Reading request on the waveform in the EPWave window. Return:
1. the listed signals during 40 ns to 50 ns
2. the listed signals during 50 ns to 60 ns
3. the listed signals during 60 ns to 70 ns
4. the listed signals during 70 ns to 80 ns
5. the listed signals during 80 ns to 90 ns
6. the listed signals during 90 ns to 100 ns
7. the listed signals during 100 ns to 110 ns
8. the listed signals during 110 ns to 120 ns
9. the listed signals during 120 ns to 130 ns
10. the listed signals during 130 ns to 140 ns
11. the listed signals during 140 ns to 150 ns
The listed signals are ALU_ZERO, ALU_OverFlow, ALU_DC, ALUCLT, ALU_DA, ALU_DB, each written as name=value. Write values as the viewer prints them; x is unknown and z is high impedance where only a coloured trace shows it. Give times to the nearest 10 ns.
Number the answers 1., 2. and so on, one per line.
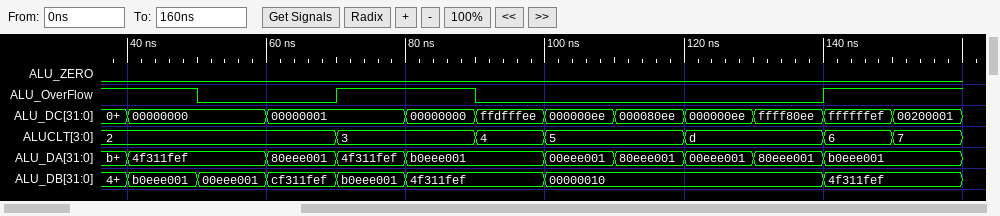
1. ALU_ZERO=0, ALU_OverFlow=1, ALU_DC=00000000, ALUCLT=2, ALU_DA=4f311fef, ALU_DB=b0eee001
2. ALU_ZERO=0, ALU_OverFlow=0, ALU_DC=00000000, ALUCLT=2, ALU_DA=4f311fef, ALU_DB=00eee001
3. ALU_ZERO=0, ALU_OverFlow=0, ALU_DC=00000001, ALUCLT=2, ALU_DA=80eee001, ALU_DB=cf311fef
4. ALU_ZERO=0, ALU_OverFlow=1, ALU_DC=00000001, ALUCLT=3, ALU_DA=4f311fef, ALU_DB=b0eee001
5. ALU_ZERO=0, ALU_OverFlow=1, ALU_DC=00000000, ALUCLT=3, ALU_DA=b0eee001, ALU_DB=4f311fef
6. ALU_ZERO=0, ALU_OverFlow=0, ALU_DC=ffdfffee, ALUCLT=4, ALU_DA=b0eee001, ALU_DB=4f311fef
7. ALU_ZERO=0, ALU_OverFlow=0, ALU_DC=000000ee, ALUCLT=5, ALU_DA=00eee001, ALU_DB=00000010
8. ALU_ZERO=0, ALU_OverFlow=0, ALU_DC=000080ee, ALUCLT=5, ALU_DA=80eee001, ALU_DB=00000010
9. ALU_ZERO=0, ALU_OverFlow=0, ALU_DC=000000ee, ALUCLT=d, ALU_DA=00eee001, ALU_DB=00000010
10. ALU_ZERO=0, ALU_OverFlow=0, ALU_DC=ffff80ee, ALUCLT=d, ALU_DA=80eee001, ALU_DB=00000010
11. ALU_ZERO=0, ALU_OverFlow=1, ALU_DC=ffffffef, ALUCLT=6, ALU_DA=b0eee001, ALU_DB=4f311fef
